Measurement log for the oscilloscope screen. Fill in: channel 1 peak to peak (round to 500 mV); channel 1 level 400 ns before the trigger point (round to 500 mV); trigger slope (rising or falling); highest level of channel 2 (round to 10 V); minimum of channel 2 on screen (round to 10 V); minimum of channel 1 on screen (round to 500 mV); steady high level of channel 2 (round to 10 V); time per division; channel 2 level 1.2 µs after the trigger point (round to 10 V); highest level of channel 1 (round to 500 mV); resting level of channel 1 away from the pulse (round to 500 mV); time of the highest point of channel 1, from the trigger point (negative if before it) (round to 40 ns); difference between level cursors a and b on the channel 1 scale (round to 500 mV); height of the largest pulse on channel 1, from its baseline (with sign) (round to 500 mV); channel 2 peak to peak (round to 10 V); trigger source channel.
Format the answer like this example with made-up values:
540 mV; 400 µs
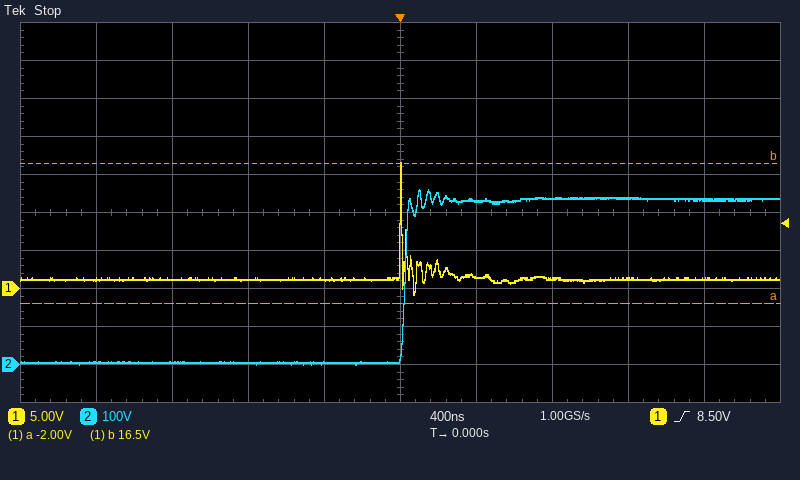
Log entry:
17.5 V; 1.0 V; rising; 460 V; 0 V; -1.0 V; 440 V; 400 ns; 440 V; 16.5 V; 1.0 V; 0 ns; 18.5 V; +15.5 V; 460 V; channel 1
